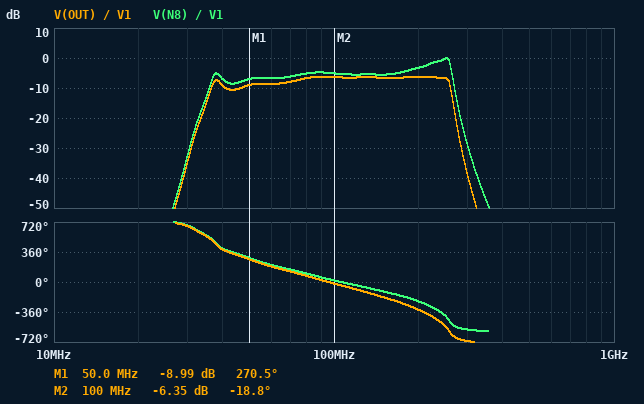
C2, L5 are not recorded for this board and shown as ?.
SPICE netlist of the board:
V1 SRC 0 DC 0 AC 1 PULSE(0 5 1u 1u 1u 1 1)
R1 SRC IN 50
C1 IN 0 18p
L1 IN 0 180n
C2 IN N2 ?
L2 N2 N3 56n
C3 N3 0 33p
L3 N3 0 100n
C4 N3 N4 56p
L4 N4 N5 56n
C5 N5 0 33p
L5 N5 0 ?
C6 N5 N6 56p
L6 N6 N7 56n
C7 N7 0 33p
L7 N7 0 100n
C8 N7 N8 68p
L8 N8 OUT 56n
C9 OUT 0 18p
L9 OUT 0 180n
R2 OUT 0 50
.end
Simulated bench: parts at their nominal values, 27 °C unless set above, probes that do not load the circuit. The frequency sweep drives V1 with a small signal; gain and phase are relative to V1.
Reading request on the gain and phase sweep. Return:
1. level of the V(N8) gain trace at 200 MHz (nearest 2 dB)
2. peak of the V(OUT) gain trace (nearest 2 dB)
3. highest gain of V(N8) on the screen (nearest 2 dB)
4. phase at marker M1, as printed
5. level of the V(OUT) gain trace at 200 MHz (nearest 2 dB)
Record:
-4 dB
-6 dB
0 dB
270.5 deg
-6 dB
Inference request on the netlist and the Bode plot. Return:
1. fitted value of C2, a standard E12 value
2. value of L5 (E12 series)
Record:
27 pF
68 nH
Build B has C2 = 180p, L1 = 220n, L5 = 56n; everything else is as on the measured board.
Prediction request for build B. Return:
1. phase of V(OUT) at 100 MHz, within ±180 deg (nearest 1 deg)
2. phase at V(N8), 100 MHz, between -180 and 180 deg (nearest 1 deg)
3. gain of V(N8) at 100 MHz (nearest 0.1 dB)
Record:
-42 deg
-4 deg
-5.2 dB
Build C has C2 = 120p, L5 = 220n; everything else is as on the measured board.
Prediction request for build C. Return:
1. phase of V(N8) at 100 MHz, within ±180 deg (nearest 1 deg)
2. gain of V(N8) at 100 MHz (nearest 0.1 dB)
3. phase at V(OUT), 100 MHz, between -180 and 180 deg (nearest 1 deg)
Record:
-30 deg
-5.1 dB
-68 deg
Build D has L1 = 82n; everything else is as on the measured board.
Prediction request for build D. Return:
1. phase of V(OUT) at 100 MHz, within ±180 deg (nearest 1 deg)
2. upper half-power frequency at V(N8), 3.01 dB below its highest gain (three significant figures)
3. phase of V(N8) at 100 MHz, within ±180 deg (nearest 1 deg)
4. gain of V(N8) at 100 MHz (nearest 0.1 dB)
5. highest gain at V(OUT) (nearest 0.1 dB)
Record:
-2 deg
260 MHz
35 deg
-4.8 dB
-6.0 dB
